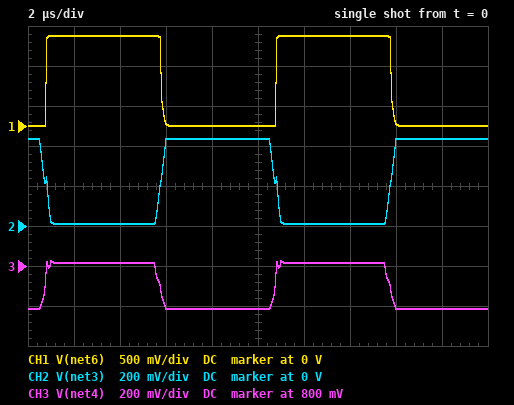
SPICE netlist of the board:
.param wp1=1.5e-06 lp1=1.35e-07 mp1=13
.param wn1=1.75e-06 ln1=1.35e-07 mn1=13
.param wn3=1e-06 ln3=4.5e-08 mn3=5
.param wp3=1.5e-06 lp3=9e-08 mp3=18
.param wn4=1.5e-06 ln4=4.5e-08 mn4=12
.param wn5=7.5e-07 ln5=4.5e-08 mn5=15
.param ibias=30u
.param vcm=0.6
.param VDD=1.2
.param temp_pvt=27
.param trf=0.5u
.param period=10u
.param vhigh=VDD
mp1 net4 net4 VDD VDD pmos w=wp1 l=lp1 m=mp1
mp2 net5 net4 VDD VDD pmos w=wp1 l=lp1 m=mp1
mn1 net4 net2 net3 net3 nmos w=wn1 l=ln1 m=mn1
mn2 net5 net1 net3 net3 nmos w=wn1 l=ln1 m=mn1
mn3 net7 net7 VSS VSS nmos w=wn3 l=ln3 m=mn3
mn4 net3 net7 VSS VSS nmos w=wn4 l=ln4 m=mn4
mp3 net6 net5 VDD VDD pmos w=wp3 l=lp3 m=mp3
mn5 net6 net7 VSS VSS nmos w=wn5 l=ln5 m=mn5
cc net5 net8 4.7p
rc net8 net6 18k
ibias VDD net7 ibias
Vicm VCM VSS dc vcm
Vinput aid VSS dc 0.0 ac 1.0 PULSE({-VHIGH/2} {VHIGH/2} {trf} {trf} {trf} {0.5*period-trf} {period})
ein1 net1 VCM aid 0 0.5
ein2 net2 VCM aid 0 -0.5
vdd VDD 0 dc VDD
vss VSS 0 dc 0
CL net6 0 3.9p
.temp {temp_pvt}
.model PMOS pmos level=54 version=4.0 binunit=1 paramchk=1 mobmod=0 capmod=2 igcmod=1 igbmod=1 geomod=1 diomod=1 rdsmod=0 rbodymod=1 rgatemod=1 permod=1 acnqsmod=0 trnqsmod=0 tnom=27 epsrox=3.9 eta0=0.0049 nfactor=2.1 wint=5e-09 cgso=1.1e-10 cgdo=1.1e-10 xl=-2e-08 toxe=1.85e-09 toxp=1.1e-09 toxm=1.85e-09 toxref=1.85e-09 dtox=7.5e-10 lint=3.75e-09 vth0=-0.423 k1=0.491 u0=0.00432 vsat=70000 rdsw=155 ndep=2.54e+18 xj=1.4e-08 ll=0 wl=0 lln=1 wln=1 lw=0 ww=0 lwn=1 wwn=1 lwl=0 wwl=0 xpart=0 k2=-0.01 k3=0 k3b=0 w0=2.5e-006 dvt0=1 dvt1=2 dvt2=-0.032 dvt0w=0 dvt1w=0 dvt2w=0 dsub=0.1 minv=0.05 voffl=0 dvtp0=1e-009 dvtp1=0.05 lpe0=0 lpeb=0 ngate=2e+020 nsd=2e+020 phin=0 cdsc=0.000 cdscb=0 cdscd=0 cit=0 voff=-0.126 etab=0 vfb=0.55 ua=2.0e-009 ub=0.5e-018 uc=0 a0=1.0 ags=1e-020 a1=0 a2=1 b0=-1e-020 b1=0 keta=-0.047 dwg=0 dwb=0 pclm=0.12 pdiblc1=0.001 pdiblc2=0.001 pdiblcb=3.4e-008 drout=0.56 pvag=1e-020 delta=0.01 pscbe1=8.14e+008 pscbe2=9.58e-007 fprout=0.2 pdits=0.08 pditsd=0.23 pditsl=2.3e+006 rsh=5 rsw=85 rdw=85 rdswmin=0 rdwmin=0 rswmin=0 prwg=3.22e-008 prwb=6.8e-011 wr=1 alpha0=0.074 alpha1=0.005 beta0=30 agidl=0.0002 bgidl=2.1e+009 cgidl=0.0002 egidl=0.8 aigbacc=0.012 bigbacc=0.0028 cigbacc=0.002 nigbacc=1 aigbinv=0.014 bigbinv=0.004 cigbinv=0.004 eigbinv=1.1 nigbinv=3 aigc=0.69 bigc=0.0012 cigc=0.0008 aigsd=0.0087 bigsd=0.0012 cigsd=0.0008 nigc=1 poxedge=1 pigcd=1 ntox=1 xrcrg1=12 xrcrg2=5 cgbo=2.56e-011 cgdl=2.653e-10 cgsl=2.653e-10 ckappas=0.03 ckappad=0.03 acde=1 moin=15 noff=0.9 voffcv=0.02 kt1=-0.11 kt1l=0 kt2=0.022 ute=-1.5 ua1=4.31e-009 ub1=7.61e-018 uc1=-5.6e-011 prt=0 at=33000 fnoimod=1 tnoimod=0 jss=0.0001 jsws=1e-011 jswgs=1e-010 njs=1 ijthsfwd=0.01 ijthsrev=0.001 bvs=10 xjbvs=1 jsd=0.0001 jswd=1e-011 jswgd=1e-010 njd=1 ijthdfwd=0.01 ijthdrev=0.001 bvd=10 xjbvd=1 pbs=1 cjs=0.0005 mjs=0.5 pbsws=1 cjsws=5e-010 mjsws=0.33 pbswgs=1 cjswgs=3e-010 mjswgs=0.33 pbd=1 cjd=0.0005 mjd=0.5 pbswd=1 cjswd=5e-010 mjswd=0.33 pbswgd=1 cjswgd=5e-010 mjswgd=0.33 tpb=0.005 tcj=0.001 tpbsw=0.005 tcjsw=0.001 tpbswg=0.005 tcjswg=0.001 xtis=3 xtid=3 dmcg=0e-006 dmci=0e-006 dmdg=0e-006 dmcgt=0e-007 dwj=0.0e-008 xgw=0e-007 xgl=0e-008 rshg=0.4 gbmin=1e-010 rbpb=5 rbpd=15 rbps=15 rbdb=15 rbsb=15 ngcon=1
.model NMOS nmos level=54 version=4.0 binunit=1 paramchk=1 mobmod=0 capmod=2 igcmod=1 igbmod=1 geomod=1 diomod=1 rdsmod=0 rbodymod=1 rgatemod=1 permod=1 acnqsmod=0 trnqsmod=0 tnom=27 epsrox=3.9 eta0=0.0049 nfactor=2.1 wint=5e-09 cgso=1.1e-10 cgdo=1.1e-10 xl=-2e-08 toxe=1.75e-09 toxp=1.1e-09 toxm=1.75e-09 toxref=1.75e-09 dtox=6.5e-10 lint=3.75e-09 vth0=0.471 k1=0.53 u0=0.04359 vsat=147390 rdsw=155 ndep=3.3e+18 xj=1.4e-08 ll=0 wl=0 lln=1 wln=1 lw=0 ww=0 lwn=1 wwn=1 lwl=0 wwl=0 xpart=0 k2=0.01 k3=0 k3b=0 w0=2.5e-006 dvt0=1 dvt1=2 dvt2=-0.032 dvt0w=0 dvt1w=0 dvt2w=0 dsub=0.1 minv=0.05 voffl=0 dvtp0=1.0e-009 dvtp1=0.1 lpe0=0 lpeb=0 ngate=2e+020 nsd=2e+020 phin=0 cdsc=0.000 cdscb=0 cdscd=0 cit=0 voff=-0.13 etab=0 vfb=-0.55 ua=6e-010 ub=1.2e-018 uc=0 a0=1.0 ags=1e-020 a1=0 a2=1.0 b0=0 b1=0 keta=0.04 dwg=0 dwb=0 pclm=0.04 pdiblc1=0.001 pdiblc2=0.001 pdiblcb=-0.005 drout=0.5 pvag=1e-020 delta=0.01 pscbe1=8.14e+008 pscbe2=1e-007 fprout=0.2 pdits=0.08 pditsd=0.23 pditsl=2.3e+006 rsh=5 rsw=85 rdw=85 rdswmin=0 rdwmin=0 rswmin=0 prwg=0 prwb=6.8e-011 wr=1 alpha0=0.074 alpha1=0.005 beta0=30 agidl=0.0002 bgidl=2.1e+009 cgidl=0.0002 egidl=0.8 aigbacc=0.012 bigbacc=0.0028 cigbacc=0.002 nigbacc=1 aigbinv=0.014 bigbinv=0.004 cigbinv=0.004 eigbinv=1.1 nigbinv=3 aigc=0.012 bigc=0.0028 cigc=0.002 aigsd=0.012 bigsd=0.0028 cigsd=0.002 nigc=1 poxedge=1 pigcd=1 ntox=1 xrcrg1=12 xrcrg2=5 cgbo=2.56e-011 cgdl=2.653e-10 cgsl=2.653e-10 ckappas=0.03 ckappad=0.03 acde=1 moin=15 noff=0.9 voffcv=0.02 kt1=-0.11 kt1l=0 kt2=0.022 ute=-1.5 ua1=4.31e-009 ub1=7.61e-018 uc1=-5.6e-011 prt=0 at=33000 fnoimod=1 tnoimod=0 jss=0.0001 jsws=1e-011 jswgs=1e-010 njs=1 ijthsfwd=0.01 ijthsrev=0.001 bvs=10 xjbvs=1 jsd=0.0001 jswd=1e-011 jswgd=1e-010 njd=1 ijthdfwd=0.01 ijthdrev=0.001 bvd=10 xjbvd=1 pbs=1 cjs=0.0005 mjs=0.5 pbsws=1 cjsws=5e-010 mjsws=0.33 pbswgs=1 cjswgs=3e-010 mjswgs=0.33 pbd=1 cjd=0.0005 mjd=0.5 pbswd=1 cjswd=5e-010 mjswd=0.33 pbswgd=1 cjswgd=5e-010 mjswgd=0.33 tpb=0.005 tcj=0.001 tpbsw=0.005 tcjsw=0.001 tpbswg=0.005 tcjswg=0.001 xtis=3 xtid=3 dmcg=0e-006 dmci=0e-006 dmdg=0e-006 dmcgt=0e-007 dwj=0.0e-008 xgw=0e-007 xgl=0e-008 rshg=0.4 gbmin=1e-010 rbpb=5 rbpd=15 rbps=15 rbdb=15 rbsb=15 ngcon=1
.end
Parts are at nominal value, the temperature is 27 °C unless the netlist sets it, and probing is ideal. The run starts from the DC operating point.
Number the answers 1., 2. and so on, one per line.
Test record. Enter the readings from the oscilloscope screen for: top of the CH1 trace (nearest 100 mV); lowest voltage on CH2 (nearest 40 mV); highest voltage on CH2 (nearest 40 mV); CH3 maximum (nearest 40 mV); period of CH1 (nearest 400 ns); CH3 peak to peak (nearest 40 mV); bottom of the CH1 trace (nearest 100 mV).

1. 1.1 V
2. 0 V
3. 440 mV
4. 840 mV
5. 10.0 µs
6. 240 mV
7. 0 V
